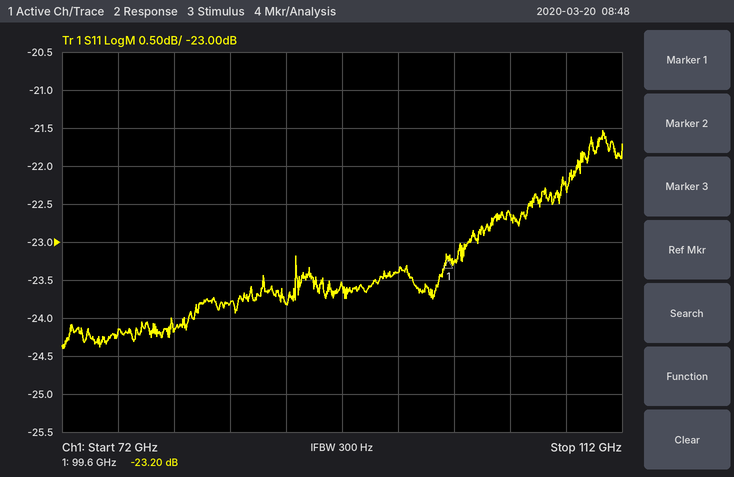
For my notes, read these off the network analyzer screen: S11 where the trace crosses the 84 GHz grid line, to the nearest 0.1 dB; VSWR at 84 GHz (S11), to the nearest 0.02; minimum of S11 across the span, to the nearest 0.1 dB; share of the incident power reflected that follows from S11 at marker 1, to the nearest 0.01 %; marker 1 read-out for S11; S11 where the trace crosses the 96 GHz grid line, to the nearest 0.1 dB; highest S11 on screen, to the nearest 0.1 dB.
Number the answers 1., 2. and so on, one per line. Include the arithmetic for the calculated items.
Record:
1. -23.8 dB
2. |Γ| = 10^(-23.8/20) = 0.0646; VSWR = (1 + 0.0646)/(1 − 0.0646) ≈ 1.14
3. -24.4 dB
4. 10^(-23.2/10) ≈ 0.48 %
5. -23.20 dB
6. -23.4 dB
7. -21.5 dB
